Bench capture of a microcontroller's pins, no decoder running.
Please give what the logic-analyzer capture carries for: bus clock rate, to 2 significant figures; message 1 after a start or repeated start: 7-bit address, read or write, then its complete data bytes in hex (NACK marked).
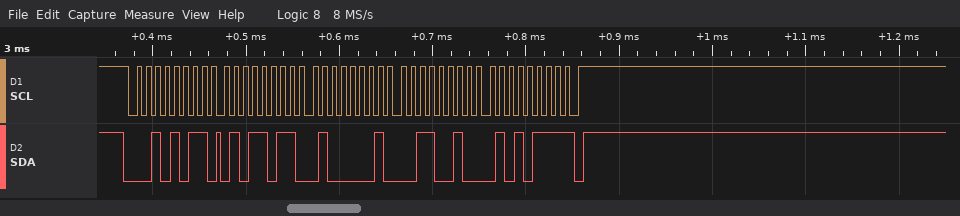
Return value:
100 kHz
0x15 read: 5B 41 32 57 NACK
